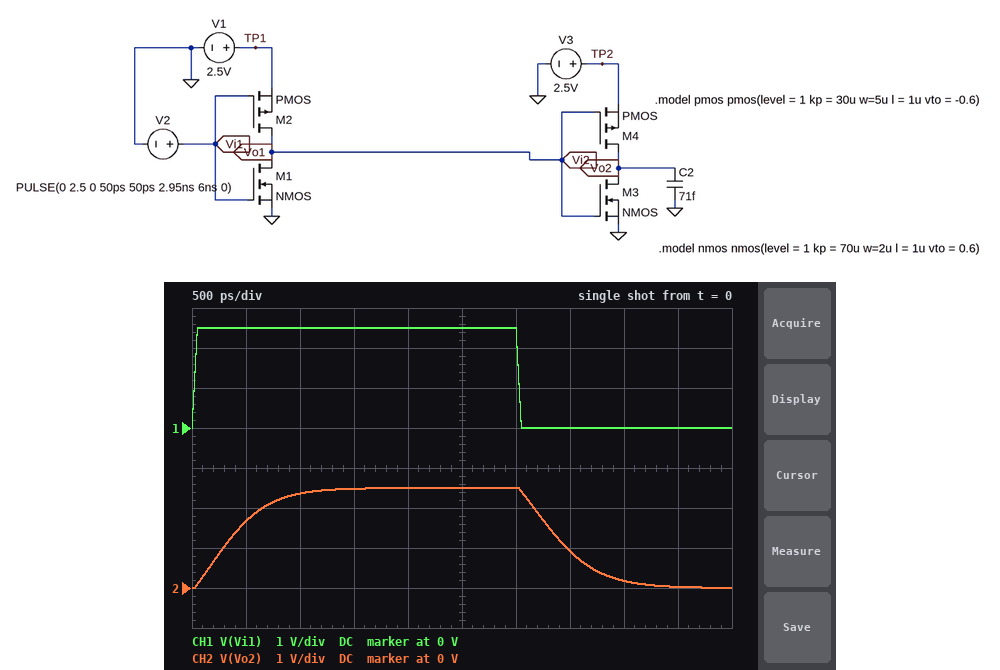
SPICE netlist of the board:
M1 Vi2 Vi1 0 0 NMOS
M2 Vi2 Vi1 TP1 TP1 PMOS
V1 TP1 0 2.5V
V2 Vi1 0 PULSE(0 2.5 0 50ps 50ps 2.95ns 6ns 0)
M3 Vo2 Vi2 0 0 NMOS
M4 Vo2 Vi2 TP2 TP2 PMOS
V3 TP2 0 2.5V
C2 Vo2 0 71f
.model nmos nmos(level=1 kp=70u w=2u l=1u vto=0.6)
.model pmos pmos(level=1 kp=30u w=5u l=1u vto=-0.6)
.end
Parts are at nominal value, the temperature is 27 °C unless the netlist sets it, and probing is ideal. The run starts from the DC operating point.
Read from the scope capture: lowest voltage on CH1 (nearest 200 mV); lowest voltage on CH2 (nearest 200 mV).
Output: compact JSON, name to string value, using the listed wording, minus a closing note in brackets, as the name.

{"lowest voltage on CH1": "0 V", "lowest voltage on CH2": "0 V"}
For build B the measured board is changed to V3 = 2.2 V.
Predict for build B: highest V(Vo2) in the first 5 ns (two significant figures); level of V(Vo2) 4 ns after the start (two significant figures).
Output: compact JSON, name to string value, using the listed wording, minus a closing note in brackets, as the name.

{"highest V(Vo2) in the first 5 ns": "2.2 V", "level of V(Vo2) 4 ns after the start": "130 mV"}
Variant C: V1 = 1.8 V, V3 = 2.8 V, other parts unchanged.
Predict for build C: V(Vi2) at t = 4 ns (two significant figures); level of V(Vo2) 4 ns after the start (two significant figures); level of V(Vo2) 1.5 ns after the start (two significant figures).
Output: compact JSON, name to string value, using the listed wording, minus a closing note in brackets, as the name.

{"V(Vi2) at t = 4 ns": "1.8 V", "level of V(Vo2) 4 ns after the start": "1.6 V", "level of V(Vo2) 1.5 ns after the start": "2.8 V"}
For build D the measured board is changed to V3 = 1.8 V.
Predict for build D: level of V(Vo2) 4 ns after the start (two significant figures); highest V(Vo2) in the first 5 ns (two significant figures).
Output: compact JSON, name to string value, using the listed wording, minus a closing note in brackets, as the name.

{"level of V(Vo2) 4 ns after the start": "87 mV", "highest V(Vo2) in the first 5 ns": "1.8 V"}
